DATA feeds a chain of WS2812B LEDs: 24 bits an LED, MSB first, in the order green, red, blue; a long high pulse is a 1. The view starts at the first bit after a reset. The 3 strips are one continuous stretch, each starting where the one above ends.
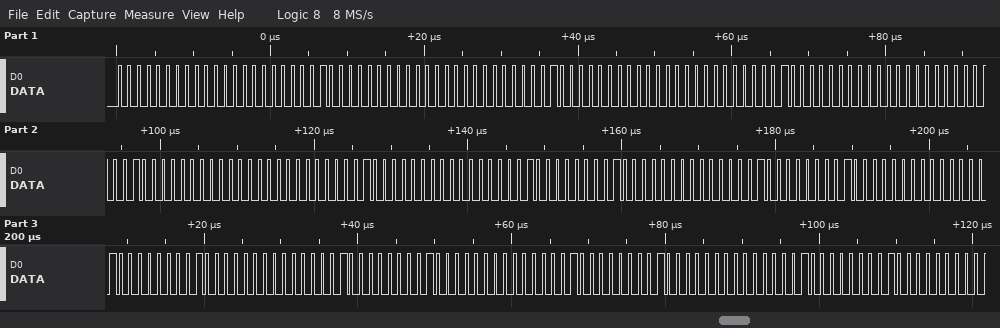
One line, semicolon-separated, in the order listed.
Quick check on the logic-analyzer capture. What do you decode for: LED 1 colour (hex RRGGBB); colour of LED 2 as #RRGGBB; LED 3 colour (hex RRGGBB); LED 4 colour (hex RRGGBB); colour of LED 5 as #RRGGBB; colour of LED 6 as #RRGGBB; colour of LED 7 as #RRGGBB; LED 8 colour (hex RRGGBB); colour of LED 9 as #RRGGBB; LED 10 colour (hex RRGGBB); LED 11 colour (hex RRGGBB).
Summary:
#000004; #000004; #000004; #000004; #000004; #020001; #020001; #020001; #020001; #020001; #020001
